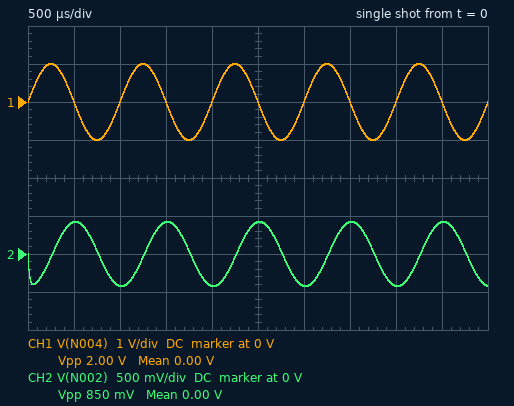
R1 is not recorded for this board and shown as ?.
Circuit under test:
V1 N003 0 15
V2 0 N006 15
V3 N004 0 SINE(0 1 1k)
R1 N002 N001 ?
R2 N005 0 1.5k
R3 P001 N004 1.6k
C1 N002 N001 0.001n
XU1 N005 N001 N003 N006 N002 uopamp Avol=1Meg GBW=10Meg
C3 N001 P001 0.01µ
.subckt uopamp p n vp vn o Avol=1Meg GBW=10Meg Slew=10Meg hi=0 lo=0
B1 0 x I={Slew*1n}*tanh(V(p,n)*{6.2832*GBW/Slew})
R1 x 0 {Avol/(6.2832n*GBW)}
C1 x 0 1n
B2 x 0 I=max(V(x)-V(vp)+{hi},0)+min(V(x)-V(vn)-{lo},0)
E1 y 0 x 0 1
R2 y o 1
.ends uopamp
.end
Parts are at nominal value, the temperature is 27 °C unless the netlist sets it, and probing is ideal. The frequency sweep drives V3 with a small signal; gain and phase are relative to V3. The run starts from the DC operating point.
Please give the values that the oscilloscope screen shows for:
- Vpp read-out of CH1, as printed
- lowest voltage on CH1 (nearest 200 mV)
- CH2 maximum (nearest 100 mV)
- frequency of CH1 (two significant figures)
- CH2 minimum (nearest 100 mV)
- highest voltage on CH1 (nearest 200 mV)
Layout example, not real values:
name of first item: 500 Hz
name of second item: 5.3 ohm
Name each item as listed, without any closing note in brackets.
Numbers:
Vpp read-out of CH1, as printed: 2.00 V
lowest voltage on CH1: -1.0 V
CH2 maximum: 400 mV
frequency of CH1: 1.0 kHz
CH2 minimum: -400 mV
highest voltage on CH1: 1.0 V
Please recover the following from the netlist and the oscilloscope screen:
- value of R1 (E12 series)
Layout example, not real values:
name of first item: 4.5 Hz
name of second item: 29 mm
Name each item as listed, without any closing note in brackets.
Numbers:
value of R1: 6.8 kΩ
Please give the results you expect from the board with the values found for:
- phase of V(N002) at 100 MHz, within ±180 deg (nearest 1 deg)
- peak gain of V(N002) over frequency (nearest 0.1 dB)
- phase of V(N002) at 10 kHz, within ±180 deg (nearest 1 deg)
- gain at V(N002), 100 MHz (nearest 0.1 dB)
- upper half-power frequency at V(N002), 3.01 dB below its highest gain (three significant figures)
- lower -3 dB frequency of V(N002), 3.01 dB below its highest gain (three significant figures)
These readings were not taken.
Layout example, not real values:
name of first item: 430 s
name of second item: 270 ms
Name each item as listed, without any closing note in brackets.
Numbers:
phase of V(N002) at 100 MHz, within ±180 deg: 54 deg
peak gain of V(N002) over frequency: 12.6 dB
phase of V(N002) at 10 kHz, within ±180 deg: -135 deg
gain at V(N002), 100 MHz: -24.3 dB
upper half-power frequency at V(N002), 3.01 dB below its highest gain: 1.80 MHz
lower -3 dB frequency of V(N002), 3.01 dB below its highest gain: 9.88 kHz
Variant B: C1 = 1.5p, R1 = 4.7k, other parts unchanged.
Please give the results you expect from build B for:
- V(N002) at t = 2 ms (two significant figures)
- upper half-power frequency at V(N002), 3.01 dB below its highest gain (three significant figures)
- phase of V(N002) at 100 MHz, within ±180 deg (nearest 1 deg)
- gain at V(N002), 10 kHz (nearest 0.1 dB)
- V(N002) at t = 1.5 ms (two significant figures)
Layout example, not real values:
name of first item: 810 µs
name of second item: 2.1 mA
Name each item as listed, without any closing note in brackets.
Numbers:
V(N002) at t = 2 ms: -290 mV
upper half-power frequency at V(N002), 3.01 dB below its highest gain: 2.35 MHz
phase of V(N002) at 100 MHz, within ±180 deg: 45 deg
gain at V(N002), 10 kHz: 6.4 dB
V(N002) at t = 1.5 ms: 290 mV
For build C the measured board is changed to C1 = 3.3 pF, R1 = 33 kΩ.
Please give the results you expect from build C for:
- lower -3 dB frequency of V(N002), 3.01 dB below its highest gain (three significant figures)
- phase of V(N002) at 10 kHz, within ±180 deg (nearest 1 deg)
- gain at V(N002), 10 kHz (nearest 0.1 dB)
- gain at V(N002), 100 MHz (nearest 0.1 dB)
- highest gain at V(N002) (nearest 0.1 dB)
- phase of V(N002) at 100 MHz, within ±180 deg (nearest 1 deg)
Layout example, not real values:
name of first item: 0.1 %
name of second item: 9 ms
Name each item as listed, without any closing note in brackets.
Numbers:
lower -3 dB frequency of V(N002), 3.01 dB below its highest gain: 9.61 kHz
phase of V(N002) at 10 kHz, within ±180 deg: -136 deg
gain at V(N002), 10 kHz: 23.4 dB
gain at V(N002), 100 MHz: -30.9 dB
highest gain at V(N002): 26.2 dB
phase of V(N002) at 100 MHz, within ±180 deg: 23 deg
